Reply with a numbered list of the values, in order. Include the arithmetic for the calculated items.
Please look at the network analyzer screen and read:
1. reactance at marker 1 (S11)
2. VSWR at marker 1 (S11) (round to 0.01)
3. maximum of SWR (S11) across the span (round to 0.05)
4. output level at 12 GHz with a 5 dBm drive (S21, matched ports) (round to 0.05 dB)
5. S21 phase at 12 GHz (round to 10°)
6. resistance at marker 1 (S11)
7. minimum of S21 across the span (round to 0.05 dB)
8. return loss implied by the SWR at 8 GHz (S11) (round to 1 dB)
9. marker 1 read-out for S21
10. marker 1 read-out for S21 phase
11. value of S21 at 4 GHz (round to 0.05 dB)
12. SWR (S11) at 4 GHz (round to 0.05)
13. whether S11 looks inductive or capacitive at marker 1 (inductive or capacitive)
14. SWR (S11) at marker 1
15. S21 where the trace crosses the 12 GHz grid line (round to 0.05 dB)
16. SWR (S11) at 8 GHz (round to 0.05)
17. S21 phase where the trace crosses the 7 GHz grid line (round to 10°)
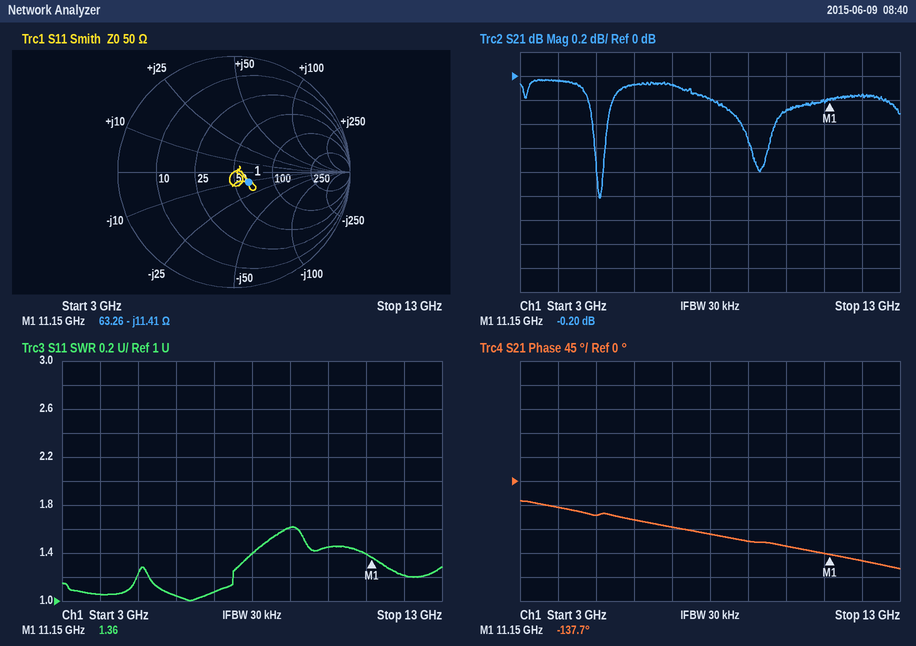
1. -11.41 Ω
2. 1.36
3. 1.60
4. 5 dBm + (-0.15 dB) = 4.85 dBm
5. -150°
6. 63.26 Ω
7. -1.00 dB
8. −20 log10((1.4 − 1)/(1.4 + 1)) ≈ 16 dB
9. -0.20 dB
10. -137.7°
11. -0.05 dB
12. 1.05
13. capacitive
14. 1.36
15. -0.15 dB
16. 1.40
17. -90°
